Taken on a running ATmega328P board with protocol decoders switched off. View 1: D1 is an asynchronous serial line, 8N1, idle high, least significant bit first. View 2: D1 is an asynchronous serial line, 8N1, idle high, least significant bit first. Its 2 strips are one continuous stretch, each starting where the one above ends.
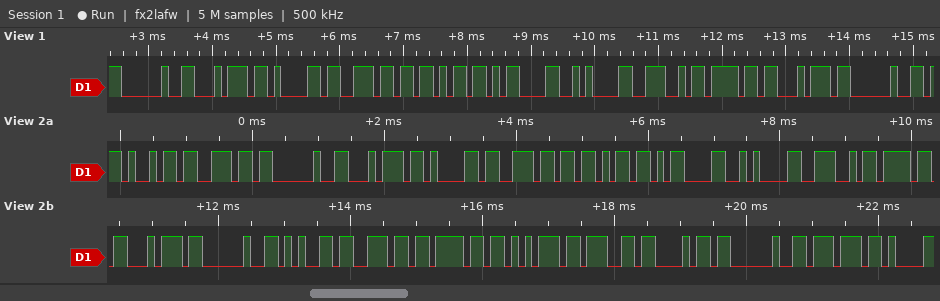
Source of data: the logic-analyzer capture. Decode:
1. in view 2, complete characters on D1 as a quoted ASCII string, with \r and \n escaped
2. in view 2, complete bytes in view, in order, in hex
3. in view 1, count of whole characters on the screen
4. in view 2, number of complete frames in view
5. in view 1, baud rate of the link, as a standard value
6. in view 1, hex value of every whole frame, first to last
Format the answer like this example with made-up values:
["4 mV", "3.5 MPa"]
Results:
["\"in tank\\r\\nNot enough w\"", "69 6E 20 74 61 6E 6B 0D 0A 4E 6F 74 20 65 6E 6F 75 67 68 20 77", "11", "21", "9600 baud", "20 74 61 6E 6B 0D 0A 4E 6F 74 20"]
